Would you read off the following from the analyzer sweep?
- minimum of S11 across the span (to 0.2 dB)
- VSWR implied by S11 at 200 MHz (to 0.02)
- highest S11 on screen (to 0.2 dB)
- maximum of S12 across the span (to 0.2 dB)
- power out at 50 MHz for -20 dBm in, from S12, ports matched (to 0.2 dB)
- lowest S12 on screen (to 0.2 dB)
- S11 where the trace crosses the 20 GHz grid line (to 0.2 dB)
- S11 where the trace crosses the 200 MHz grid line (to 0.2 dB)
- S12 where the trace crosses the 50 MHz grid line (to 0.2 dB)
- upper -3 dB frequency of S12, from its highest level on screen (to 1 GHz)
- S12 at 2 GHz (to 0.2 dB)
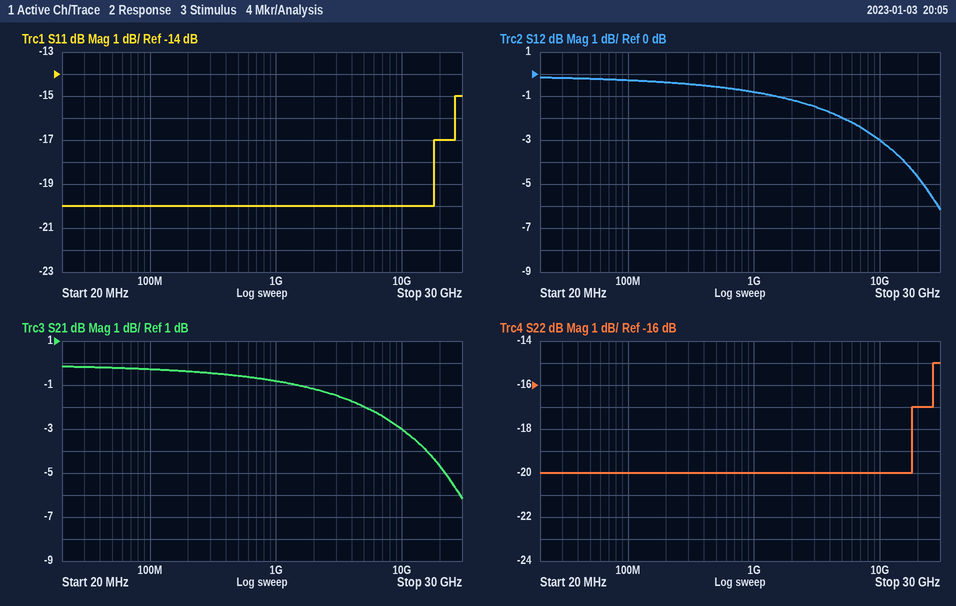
-20.0 dB
1.22
-15.0 dB
-0.2 dB
-20.2 dBm
-6.2 dB
-17.0 dB
-20.0 dB
-0.2 dB
11 GHz
-1.2 dB
